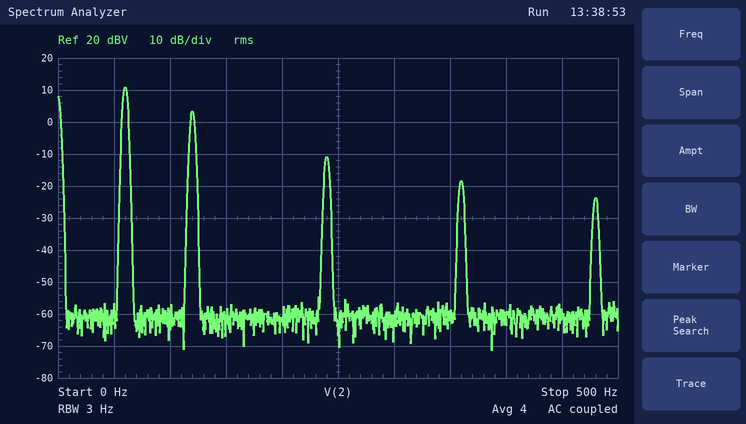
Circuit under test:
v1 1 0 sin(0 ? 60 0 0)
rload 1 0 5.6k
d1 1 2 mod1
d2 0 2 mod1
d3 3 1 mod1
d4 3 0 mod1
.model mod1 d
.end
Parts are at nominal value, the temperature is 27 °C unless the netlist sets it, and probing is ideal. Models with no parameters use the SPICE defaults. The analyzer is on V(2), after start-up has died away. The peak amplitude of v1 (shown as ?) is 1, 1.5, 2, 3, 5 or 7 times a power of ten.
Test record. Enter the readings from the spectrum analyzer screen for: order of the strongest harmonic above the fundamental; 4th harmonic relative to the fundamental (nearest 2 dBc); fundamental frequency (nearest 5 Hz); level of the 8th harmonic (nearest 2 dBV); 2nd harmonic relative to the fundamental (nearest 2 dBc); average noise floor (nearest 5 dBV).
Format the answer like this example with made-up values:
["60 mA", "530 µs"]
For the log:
["2", "-22 dBc", "60 Hz", "-24 dBV", "-8 dBc", "-60 dBV"]
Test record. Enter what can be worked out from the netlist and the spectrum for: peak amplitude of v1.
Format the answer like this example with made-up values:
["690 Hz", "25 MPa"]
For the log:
["10 V"]
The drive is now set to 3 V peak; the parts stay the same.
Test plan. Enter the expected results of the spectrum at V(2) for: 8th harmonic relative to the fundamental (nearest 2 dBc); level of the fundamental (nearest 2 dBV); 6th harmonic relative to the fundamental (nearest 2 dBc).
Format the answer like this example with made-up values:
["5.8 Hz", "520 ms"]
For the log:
["-36 dBc", "0 dBV", "-30 dBc"]
